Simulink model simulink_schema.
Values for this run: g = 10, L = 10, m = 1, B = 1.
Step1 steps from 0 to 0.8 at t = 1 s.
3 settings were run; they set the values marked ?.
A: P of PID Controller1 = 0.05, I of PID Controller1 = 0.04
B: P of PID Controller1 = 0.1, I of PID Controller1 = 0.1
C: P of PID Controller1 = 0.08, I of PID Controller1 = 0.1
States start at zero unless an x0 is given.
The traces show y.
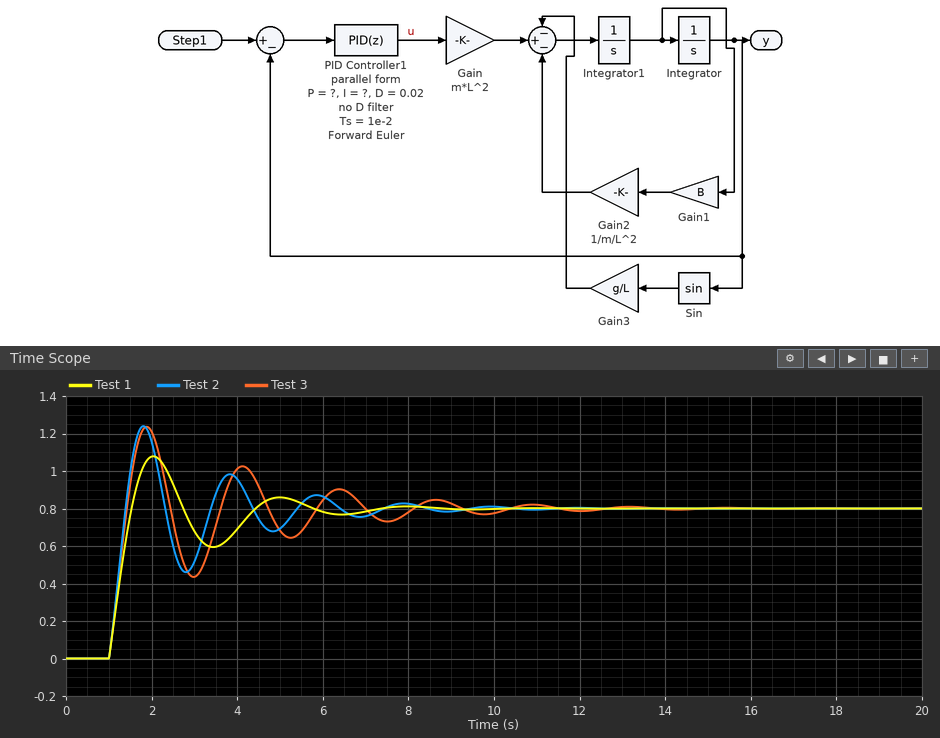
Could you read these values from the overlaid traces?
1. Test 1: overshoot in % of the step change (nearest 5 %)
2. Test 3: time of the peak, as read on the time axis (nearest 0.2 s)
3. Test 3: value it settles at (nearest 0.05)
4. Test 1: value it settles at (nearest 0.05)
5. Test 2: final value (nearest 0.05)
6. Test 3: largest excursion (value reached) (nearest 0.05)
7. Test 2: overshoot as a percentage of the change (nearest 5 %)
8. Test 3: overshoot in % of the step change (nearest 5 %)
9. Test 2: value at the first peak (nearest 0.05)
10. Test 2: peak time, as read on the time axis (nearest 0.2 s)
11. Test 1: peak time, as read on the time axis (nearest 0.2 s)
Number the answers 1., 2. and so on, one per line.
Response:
1. 35 %
2. 1.8 s
3. 0.80
4. 0.80
5. 0.80
6. 1.25
7. 55 %
8. 55 %
9. 1.25
10. 1.8 s
11. 2.0 s
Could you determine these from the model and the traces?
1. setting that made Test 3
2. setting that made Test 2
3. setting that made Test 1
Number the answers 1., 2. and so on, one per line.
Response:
1. C
2. B
3. A
